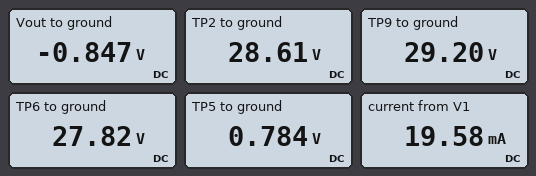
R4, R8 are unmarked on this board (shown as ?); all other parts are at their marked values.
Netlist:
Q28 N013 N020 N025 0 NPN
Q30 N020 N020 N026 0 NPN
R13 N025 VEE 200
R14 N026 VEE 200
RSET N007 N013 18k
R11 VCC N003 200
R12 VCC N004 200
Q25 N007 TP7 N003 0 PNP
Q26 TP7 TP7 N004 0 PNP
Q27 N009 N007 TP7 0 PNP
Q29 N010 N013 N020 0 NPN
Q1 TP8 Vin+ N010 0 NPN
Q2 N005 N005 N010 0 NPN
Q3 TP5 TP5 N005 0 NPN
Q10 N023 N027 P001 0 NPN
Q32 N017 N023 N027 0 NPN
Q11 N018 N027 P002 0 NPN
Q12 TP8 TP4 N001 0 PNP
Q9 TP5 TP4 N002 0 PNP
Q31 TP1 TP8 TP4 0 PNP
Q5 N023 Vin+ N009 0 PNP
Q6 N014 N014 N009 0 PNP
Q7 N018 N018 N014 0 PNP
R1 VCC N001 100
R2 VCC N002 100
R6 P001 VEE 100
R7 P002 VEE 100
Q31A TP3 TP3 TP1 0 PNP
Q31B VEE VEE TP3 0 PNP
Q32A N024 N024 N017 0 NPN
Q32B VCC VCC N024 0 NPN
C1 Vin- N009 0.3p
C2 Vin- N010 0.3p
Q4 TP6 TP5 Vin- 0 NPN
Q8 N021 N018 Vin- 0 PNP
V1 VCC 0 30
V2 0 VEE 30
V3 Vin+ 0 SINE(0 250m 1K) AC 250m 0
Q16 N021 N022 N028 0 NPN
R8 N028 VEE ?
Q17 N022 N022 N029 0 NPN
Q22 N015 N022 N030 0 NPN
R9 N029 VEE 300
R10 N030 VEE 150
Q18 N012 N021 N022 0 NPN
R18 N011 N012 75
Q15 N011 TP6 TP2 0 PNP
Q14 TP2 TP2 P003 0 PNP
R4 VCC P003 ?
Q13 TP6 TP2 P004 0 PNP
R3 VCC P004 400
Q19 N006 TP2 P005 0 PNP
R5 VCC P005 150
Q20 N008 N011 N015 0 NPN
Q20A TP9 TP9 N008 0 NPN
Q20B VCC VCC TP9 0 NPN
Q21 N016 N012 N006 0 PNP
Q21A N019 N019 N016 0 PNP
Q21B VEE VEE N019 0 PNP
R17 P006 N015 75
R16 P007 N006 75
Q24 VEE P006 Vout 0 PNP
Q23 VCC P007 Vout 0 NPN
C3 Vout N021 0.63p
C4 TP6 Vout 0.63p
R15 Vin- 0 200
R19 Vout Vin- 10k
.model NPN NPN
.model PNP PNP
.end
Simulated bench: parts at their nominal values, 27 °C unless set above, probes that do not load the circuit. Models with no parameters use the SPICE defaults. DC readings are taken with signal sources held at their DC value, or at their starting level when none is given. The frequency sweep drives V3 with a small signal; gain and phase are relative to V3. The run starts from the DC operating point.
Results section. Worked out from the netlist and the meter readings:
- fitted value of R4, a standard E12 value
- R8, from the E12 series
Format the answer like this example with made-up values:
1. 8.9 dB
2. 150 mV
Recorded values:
1. 390 Ω
2. 330 Ω
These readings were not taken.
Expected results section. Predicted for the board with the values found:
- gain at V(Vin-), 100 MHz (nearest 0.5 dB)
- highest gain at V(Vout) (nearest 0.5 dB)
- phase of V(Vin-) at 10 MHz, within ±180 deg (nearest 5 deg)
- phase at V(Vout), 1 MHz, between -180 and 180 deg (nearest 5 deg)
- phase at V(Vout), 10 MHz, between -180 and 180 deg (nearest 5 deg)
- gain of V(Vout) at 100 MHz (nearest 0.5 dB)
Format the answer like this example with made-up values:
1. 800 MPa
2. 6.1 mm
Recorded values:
1. -0.5 dB
2. 34.0 dB
3. 0 deg
4. -5 deg
5. -40 deg
6. 15.5 dB
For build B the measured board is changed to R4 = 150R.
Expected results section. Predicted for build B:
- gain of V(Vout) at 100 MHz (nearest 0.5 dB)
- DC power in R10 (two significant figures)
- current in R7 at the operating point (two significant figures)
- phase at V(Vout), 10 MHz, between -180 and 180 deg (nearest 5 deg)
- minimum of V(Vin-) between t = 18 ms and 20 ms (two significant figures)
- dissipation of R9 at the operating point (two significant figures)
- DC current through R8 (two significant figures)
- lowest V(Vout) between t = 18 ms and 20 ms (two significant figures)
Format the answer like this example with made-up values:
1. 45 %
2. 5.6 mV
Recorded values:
1. 14.5 dB
2. 3.3 mW
3. 1.6 mA
4. -45 deg
5. -240 mV
6. 1.7 mW
7. 2.2 mA
8. -100 mV
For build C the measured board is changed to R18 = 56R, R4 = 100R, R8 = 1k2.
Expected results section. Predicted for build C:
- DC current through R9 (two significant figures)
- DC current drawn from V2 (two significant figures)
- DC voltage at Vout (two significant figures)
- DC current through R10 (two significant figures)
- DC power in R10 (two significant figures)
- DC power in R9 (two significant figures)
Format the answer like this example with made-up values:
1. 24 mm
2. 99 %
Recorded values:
1. 5.5 mA
2. 31 mA
3. -960 mV
4. 11 mA
5. 18 mW
6. 9.0 mW
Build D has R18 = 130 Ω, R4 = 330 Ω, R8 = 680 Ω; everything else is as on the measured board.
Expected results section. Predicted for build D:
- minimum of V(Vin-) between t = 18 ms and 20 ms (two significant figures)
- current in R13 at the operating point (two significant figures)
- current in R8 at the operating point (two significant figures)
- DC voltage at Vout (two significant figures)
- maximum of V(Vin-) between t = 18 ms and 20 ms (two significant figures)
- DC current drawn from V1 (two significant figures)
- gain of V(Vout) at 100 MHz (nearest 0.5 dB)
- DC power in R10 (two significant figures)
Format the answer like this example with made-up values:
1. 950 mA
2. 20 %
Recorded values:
1. -260 mV
2. 3.1 mA
3. 1.1 mA
4. -9.3 V
5. 240 mV
6. 23 mA
7. 15.0 dB
8. 3.3 mW
